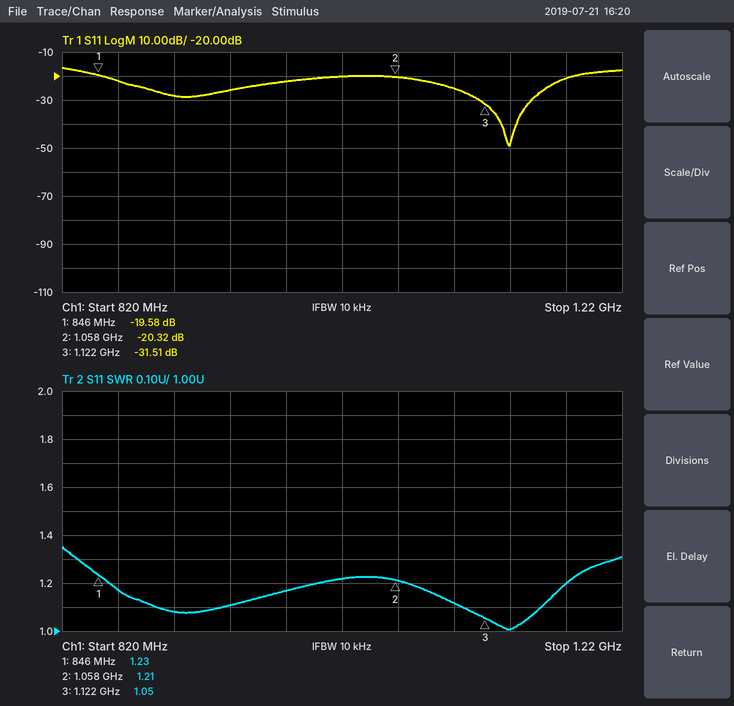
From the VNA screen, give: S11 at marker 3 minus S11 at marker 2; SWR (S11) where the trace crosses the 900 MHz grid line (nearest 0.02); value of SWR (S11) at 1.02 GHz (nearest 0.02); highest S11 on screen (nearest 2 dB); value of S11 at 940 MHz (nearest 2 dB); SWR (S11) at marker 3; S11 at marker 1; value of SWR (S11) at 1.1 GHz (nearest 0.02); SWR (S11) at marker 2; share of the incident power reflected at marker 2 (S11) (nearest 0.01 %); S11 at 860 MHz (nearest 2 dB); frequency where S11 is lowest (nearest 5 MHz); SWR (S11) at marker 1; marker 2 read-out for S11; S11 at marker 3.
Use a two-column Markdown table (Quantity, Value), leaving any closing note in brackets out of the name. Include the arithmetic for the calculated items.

| Quantity | Value |
|---|---|
| S11 at marker 3 minus S11 at marker 2 | -31.51 − (-20.32) = -11.19 dB |
| SWR (S11) where the trace crosses the 900 MHz grid line | 1.08 |
| value of SWR (S11) at 1.02 GHz | 1.22 |
| highest S11 on screen | -16 dB |
| value of S11 at 940 MHz | -26 dB |
| SWR (S11) at marker 3 | 1.05 |
| S11 at marker 1 | -19.58 dB |
| value of SWR (S11) at 1.1 GHz | 1.12 |
| SWR (S11) at marker 2 | 1.21 |
| share of the incident power reflected at marker 2 (S11) | 10^(-20.32/10) ≈ 0.93 % |
| S11 at 860 MHz | -22 dB |
| frequency where S11 is lowest | 1.140 GHz |
| SWR (S11) at marker 1 | 1.23 |
| marker 2 read-out for S11 | -20.32 dB |
| S11 at marker 3 | -31.51 dB |
